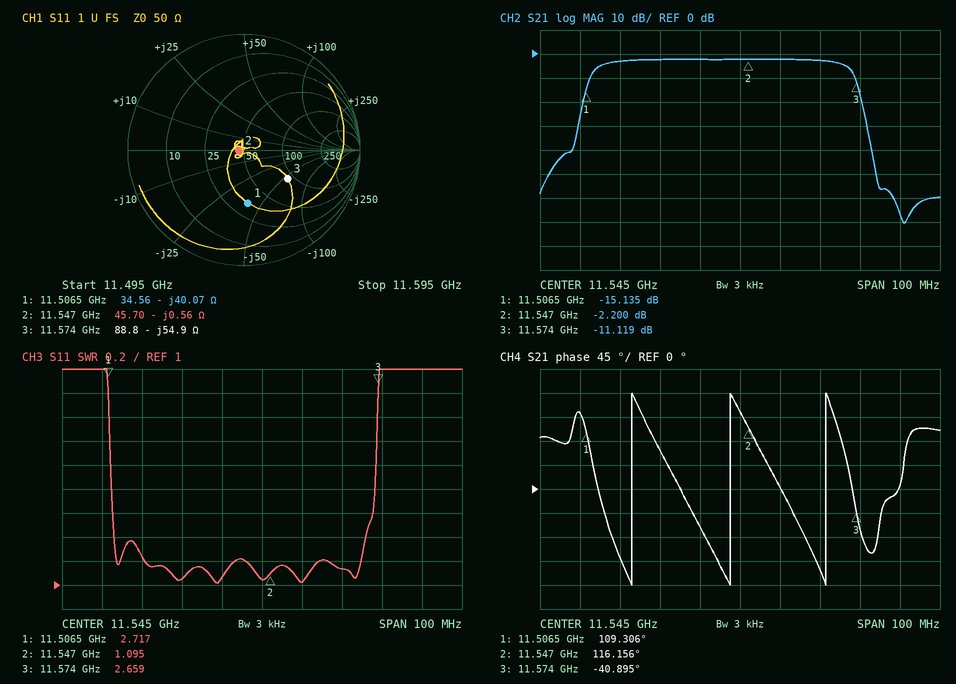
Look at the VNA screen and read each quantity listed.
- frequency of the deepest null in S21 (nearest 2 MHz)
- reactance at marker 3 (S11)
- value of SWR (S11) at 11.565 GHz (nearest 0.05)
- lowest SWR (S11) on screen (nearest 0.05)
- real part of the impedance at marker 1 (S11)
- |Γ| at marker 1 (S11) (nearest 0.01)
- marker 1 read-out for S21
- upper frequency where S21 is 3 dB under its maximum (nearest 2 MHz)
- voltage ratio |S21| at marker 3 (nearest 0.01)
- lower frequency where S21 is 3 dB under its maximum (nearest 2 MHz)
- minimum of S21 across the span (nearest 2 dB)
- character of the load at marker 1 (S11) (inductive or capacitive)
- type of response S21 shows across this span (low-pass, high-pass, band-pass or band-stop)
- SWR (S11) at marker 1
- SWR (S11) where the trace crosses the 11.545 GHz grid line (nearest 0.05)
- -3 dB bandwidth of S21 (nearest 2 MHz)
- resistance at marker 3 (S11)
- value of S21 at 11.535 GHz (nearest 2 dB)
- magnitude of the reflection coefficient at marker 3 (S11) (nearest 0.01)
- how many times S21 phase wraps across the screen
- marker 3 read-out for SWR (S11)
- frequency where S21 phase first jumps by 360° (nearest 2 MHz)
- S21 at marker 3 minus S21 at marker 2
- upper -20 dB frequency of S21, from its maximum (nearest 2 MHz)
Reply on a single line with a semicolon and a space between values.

11.586 GHz; -54.9 Ω; 1.15; 1.00; 34.56 Ω; 0.46; -15.135 dB; 11.572 GHz; 0.28; 11.510 GHz; -70 dB; capacitive; band-pass; 2.717; 1.05; 62 MHz; 88.8 Ω; -2 dB; 0.45; 3; 2.659; 11.518 GHz; -8.919 dB; 11.576 GHz
